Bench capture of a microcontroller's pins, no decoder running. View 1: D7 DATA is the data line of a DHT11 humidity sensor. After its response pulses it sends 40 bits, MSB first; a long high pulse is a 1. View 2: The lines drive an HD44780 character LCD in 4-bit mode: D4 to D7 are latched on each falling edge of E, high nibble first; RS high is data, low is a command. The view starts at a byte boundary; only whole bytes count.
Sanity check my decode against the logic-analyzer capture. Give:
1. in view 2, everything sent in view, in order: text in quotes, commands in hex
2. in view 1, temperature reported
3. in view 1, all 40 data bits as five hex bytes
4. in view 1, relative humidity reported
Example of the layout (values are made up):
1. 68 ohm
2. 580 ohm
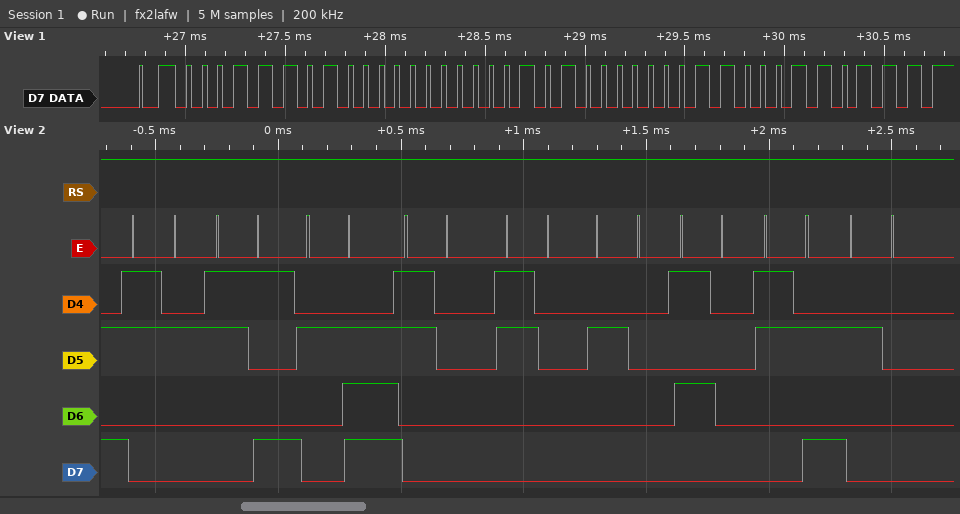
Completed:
1. "29.00 P: "
2. 20.6 °C
3. 1D 00 14 06 37
4. 29 %
